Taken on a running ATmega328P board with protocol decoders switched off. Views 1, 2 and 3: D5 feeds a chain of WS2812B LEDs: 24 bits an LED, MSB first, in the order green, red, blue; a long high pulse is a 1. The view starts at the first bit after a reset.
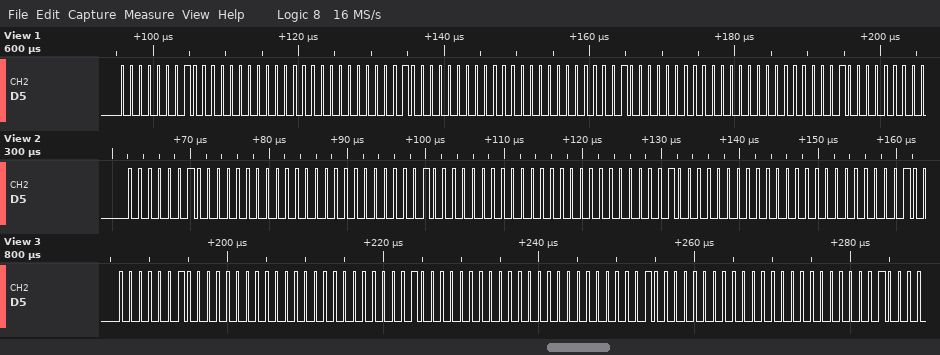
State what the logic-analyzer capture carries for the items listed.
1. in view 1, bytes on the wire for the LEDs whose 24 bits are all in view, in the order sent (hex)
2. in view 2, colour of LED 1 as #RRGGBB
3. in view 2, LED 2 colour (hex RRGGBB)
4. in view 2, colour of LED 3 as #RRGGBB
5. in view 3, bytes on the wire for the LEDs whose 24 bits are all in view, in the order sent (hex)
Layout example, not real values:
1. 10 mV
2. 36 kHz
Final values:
1. 01 00 00 01 00 00 01 00 00
2. #000200
3. #000200
4. #000100
5. 02 00 00 02 00 00 02 00 00
